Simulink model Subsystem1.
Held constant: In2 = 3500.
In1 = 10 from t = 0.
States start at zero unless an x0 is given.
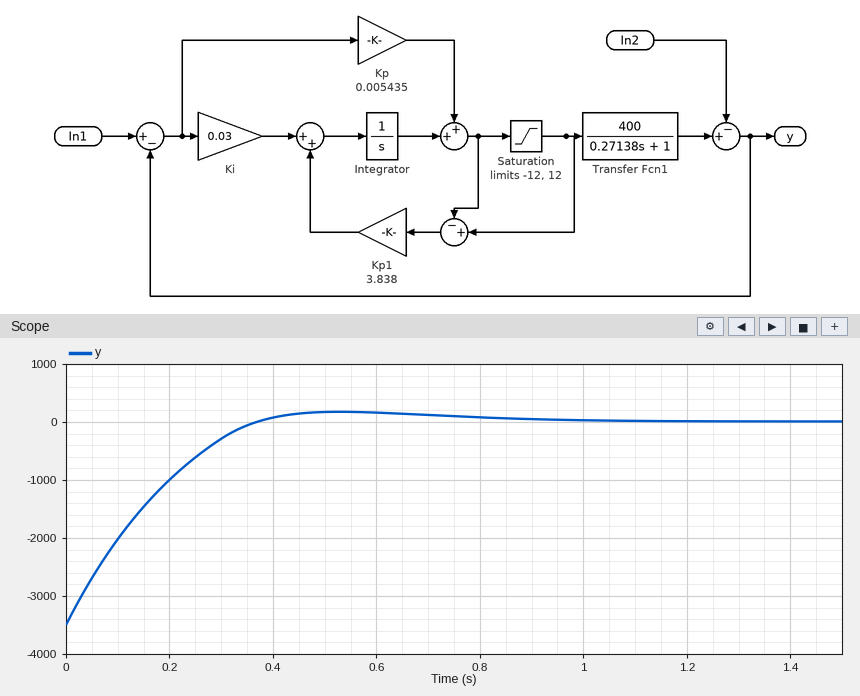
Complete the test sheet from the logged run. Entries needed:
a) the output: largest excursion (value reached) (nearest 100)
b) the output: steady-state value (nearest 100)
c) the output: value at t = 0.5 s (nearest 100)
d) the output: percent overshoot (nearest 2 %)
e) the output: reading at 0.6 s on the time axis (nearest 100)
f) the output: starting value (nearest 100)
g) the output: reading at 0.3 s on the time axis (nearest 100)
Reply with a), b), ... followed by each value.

a) 200
b) 0
c) 200
d) 4 %
e) 200
f) -3500
g) -300
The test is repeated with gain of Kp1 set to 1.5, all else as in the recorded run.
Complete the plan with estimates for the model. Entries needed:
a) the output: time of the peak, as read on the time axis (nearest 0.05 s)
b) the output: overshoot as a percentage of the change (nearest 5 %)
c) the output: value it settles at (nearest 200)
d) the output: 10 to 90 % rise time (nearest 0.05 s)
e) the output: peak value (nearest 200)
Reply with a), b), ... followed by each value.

a) 0.50 s
b) 10 %
c) 0
d) 0.25 s
e) 400
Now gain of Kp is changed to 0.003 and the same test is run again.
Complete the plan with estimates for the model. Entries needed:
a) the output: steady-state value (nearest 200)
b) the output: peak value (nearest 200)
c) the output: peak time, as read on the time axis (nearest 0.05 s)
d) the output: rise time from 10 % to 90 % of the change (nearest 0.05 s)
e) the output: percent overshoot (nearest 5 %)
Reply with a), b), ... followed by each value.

a) 0
b) 400
c) 0.55 s
d) 0.25 s
e) 10 %
